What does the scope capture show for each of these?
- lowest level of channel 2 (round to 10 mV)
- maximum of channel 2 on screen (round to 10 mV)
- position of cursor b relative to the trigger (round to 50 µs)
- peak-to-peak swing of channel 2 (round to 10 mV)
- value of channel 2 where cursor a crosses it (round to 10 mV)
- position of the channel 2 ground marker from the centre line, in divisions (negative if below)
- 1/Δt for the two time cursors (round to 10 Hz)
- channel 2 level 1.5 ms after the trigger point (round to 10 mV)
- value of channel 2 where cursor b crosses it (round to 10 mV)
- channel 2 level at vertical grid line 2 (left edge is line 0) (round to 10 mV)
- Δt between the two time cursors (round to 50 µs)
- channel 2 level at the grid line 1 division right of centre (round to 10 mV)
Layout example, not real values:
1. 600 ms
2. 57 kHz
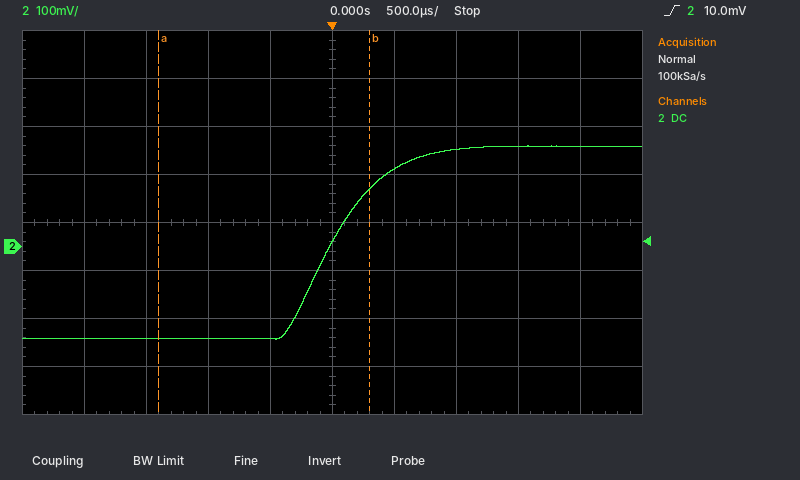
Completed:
1. -190 mV
2. 210 mV
3. +300 µs
4. 400 mV
5. -190 mV
6. -0.5 div
7. 590 Hz
8. 210 mV
9. 120 mV
10. -190 mV
11. 1.70 ms
12. 160 mV
